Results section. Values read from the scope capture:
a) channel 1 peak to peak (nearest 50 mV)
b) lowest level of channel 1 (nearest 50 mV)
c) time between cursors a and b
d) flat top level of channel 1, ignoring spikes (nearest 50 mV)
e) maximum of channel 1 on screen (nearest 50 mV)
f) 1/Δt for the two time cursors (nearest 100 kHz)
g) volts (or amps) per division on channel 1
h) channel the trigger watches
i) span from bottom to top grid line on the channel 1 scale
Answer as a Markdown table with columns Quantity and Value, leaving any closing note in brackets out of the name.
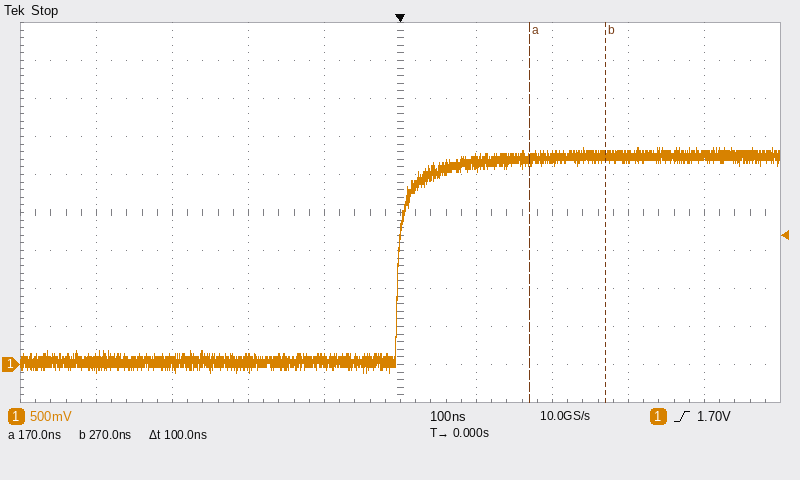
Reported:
| Quantity | Value |
|---|---|
| channel 1 peak to peak | 2.95 V |
| lowest level of channel 1 | -100 mV |
| time between cursors a and b | 100 ns |
| flat top level of channel 1, ignoring spikes | 2.75 V |
| maximum of channel 1 on screen | 2.85 V |
| 1/Δt for the two time cursors | 10.0 MHz |
| volts (or amps) per division on channel 1 | 500 mV |
| channel the trigger watches | channel 1 |
| span from bottom to top grid line on the channel 1 scale | 5 V |
